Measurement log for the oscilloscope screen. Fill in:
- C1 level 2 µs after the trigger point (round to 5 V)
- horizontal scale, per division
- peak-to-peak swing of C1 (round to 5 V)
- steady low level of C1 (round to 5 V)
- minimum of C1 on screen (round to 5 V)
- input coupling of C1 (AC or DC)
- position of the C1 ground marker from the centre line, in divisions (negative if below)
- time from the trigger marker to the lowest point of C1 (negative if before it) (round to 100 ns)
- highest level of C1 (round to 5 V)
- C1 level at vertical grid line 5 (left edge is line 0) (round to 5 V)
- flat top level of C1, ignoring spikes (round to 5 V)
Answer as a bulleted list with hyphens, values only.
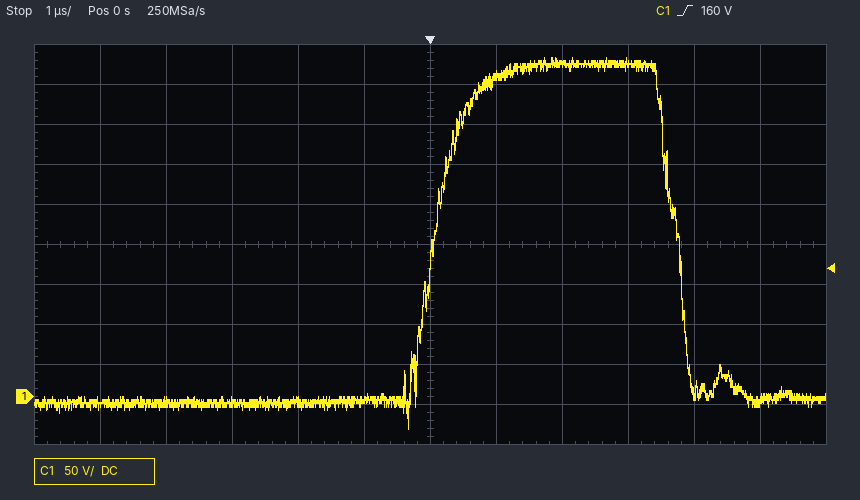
- 415 V
- 1 µs
- 465 V
- -10 V
- -40 V
- DC
- -3.8 div
- -300 ns
- 425 V
- -5 V
- 415 V
